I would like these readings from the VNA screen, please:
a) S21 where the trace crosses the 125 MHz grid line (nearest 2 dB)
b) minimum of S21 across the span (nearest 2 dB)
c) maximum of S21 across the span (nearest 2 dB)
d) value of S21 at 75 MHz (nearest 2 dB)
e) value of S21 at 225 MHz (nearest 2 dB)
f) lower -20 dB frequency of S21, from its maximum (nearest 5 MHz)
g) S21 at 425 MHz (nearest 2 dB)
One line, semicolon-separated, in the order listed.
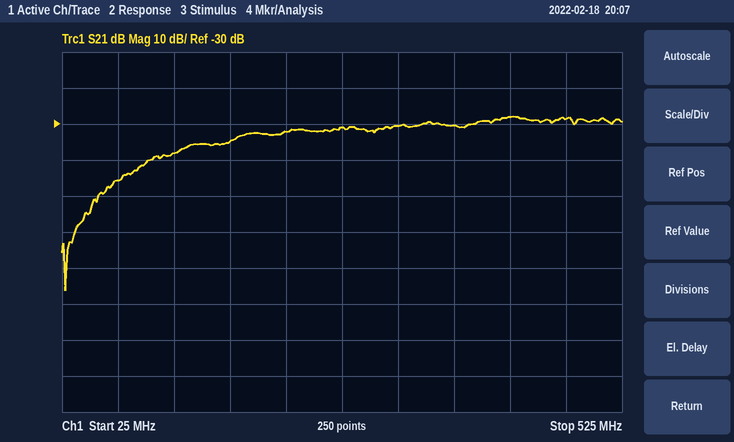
-38 dB; -76 dB; -28 dB; -46 dB; -32 dB; 65 MHz; -28 dB
